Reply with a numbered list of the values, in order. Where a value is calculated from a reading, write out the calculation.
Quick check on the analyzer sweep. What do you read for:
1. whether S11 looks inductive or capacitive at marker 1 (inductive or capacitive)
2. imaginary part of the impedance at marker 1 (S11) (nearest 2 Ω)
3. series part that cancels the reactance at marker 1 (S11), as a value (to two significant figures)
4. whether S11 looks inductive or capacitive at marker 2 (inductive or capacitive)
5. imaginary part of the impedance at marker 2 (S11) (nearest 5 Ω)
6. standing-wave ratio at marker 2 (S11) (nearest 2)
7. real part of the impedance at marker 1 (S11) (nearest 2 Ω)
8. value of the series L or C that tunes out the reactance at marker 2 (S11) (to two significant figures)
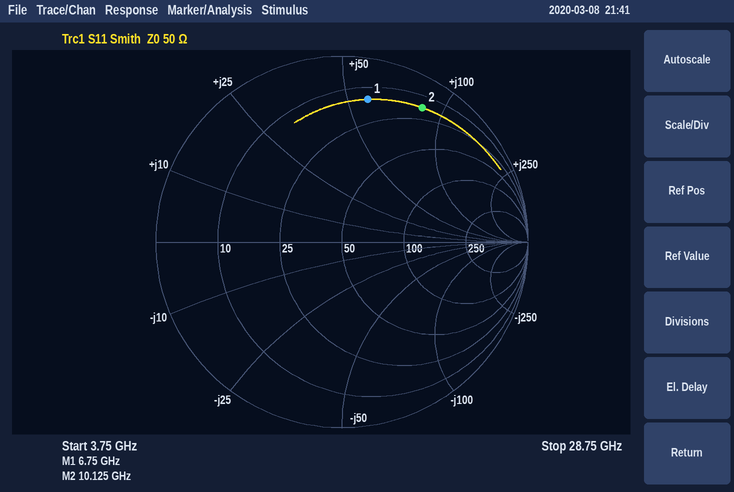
1. inductive
2. +58 Ω
3. C = 1/(2π × 6.75 GHz × 58 Ω) ≈ 407 fF, so 410 fF to two significant figures
4. inductive
5. +85 Ω
6. 12
7. 14 Ω
8. C = 1/(2π × 10.125 GHz × 85 Ω) ≈ 185 fF, so 180 fF to two significant figures
